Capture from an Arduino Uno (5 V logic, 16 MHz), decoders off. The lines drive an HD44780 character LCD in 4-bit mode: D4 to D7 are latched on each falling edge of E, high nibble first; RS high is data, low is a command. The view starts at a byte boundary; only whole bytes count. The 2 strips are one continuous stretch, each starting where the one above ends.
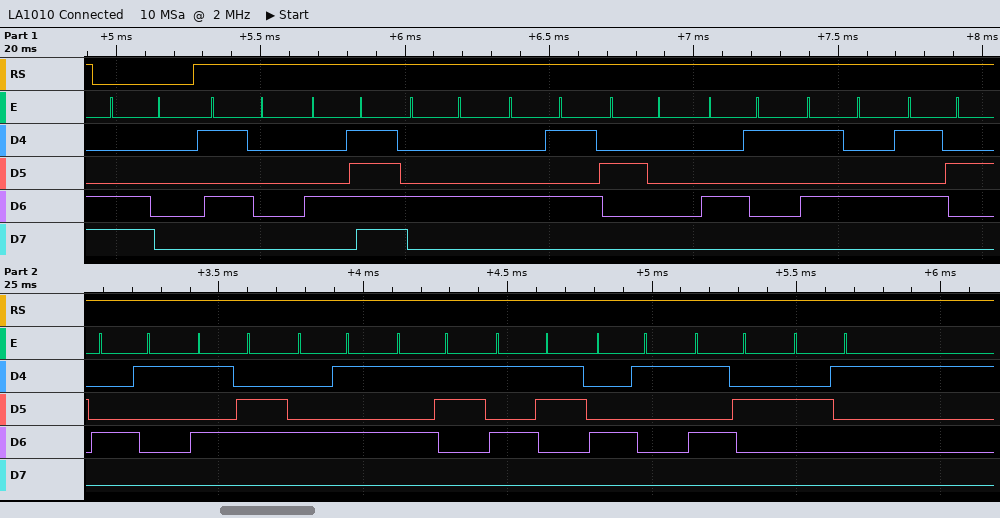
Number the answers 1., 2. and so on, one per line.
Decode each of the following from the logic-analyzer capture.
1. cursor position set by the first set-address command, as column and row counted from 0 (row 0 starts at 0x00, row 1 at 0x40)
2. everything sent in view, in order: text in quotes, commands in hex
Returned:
1. column 0, row 1
2. 0xC0 "PODE ATRAVESSAR!"
